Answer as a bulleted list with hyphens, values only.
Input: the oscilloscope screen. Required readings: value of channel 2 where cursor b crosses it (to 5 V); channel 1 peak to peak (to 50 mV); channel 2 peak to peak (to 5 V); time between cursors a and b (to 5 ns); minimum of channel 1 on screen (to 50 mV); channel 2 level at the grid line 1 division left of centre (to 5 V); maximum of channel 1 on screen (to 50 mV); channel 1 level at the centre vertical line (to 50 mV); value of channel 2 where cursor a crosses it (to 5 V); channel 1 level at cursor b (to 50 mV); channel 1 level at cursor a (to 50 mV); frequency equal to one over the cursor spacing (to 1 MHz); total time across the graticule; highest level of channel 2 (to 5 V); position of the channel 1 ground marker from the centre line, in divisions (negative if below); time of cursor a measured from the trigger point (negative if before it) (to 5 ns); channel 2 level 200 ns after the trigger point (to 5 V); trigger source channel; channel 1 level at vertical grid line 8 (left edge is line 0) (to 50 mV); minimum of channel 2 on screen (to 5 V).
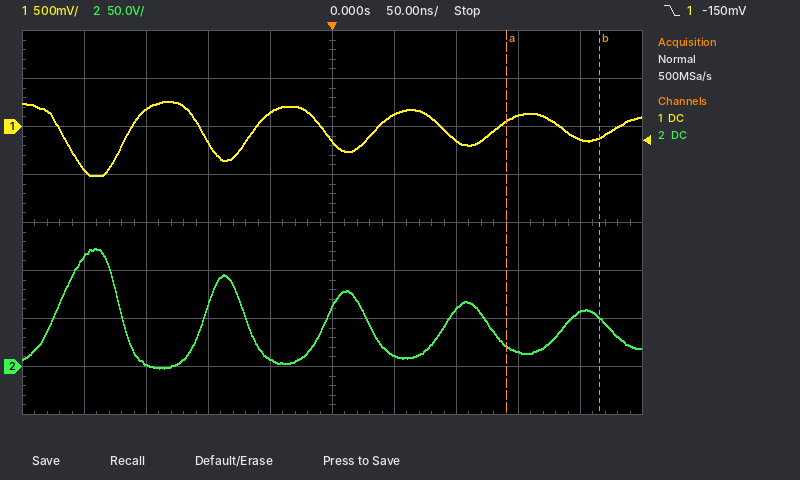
- 50 V
- 750 mV
- 125 V
- 75 ns
- -500 mV
- 10 V
- 250 mV
- -150 mV
- 20 V
- -100 mV
- 50 mV
- 13 MHz
- 500 ns
- 125 V
- +2.0 div
- +140 ns
- 55 V
- channel 1
- 100 mV
- 0 V
